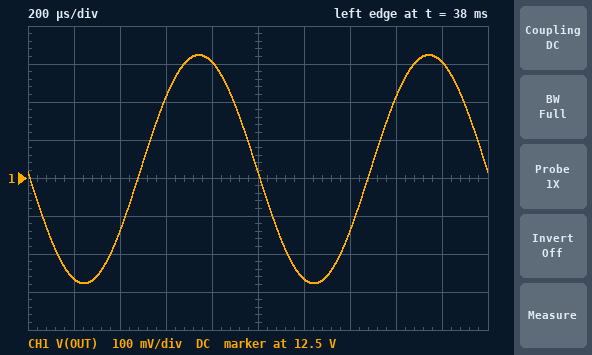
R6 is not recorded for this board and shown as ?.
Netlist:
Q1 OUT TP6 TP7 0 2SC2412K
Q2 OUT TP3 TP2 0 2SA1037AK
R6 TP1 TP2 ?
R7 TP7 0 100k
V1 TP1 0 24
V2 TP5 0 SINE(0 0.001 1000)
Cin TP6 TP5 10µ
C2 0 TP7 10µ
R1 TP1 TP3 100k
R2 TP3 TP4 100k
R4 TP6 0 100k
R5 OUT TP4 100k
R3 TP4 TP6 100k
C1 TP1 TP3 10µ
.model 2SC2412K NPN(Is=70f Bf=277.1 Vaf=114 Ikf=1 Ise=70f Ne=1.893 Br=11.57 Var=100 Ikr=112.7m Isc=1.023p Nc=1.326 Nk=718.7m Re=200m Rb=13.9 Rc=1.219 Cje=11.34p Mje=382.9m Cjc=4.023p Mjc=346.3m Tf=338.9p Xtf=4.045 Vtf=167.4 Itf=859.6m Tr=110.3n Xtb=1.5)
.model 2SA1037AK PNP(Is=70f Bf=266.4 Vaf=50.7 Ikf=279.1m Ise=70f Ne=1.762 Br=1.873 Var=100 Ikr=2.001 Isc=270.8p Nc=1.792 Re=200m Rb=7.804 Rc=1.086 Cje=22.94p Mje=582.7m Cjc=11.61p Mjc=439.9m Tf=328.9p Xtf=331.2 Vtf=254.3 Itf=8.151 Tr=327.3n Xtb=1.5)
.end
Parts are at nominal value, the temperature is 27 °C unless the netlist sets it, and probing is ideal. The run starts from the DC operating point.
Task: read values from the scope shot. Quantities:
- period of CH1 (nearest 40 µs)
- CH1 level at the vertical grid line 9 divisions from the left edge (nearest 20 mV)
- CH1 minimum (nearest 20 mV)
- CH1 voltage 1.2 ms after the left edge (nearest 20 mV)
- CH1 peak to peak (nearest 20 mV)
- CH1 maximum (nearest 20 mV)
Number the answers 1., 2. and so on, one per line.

1. 1.00 ms
2. 12.80 V
3. 12.22 V
4. 12.24 V
5. 600 mV
6. 12.82 V
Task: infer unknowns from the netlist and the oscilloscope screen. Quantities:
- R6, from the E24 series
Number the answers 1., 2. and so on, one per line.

1. 91 kΩ
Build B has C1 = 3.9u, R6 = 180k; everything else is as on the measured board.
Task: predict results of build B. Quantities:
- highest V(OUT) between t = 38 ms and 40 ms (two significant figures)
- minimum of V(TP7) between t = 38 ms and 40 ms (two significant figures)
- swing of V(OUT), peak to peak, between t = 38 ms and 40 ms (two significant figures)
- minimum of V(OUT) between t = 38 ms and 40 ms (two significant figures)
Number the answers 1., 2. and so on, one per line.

1. 9.5 V
2. 4.8 V
3. 520 mV
4. 9.0 V
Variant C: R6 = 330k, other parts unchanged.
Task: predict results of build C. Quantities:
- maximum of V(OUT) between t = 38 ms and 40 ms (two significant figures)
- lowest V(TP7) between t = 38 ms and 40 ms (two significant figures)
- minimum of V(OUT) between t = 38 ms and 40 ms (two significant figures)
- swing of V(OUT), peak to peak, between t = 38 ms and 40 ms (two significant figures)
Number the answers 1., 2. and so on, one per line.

1. 7.6 V
2. 4.3 V
3. 7.2 V
4. 470 mV
